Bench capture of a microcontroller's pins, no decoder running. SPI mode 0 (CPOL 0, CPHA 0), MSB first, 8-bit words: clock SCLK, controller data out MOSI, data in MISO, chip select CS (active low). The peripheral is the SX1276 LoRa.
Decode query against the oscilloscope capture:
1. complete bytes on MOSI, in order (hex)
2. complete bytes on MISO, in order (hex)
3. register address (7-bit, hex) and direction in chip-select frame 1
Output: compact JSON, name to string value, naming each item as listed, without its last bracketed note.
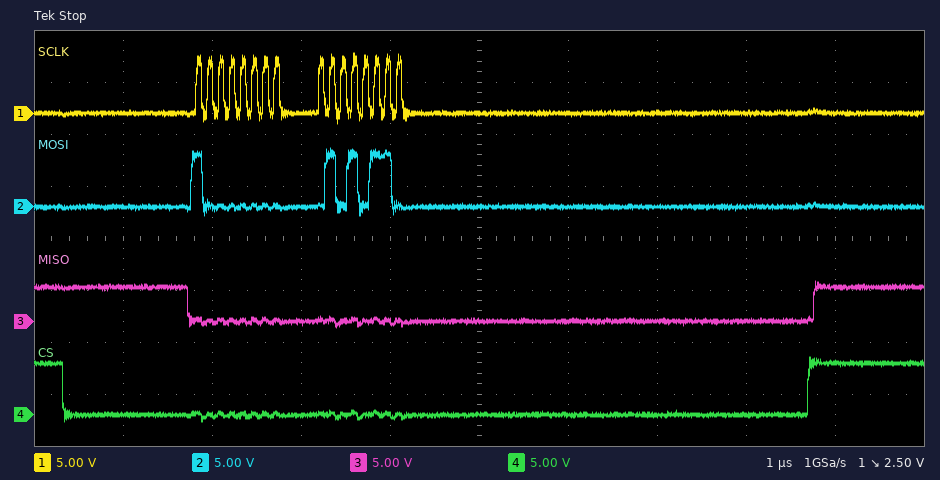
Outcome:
{"complete bytes on MOSI, in order": "80 56", "complete bytes on MISO, in order": "00 00", "register address (7-bit, hex) and direction in chip-select frame 1": "0x00 write"}
